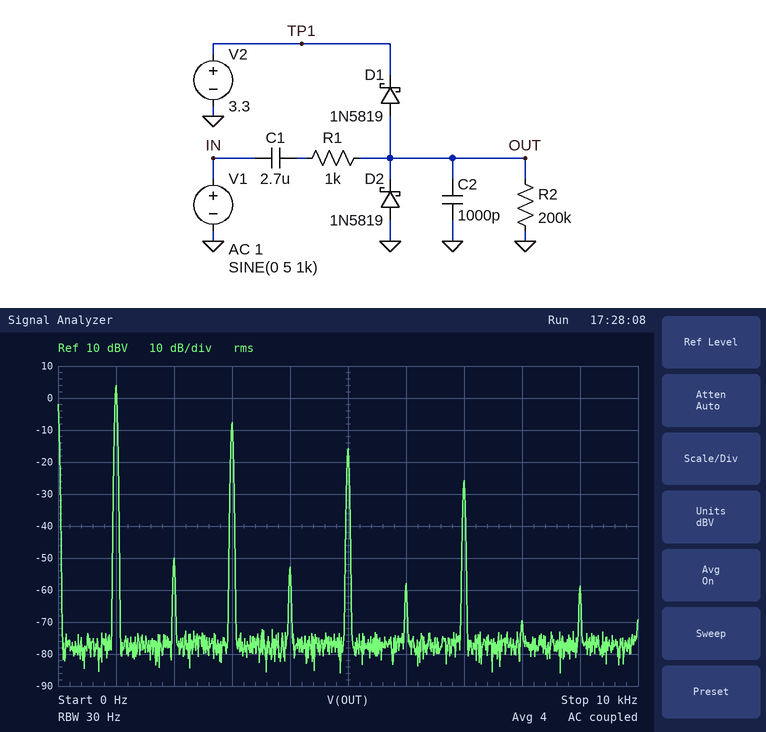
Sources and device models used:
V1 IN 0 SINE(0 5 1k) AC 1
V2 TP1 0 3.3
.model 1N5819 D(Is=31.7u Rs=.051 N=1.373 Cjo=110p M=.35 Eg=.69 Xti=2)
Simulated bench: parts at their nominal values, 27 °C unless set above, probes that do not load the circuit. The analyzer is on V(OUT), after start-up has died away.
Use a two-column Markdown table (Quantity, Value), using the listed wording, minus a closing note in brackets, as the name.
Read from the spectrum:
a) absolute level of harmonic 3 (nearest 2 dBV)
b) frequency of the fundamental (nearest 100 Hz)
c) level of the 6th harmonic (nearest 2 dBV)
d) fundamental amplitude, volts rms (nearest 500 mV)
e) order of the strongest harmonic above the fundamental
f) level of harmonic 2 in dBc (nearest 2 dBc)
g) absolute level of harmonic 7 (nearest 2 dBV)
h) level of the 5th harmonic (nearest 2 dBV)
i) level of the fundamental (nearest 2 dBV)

| Quantity | Value |
|---|---|
| absolute level of harmonic 3 | -8 dBV |
| frequency of the fundamental | 1.0 kHz |
| level of the 6th harmonic | -58 dBV |
| fundamental amplitude, volts rms | 1.5 V |
| order of the strongest harmonic above the fundamental | 3 |
| level of harmonic 2 in dBc | -54 dBc |
| absolute level of harmonic 7 | -26 dBV |
| level of the 5th harmonic | -16 dBV |
| level of the fundamental | 4 dBV |
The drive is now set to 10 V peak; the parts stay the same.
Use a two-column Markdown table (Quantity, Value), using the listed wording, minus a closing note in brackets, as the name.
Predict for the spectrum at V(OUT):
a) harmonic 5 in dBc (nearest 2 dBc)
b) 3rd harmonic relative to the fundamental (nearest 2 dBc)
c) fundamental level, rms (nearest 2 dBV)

| Quantity | Value |
|---|---|
| harmonic 5 in dBc | -16 dBc |
| 3rd harmonic relative to the fundamental | -10 dBc |
| fundamental level, rms | 4 dBV |
